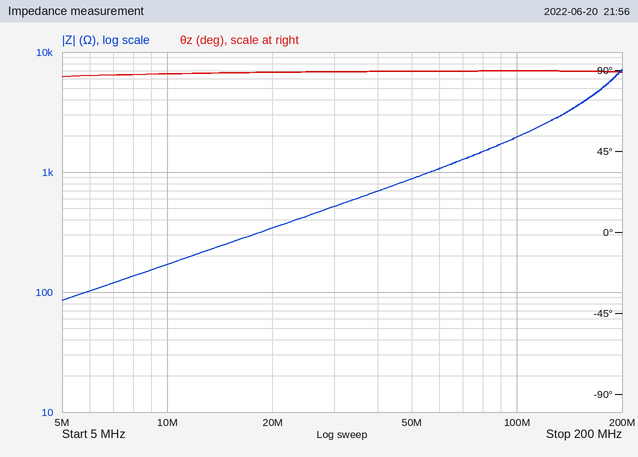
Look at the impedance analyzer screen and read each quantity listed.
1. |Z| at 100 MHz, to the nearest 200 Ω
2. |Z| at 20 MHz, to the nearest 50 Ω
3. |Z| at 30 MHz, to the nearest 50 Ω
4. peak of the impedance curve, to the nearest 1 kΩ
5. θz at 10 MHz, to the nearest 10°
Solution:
2.0 kΩ
350 Ω
500 Ω
7 kΩ
90°
